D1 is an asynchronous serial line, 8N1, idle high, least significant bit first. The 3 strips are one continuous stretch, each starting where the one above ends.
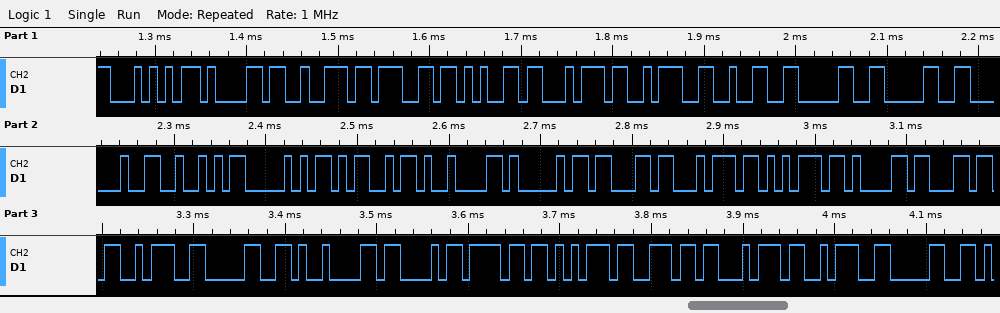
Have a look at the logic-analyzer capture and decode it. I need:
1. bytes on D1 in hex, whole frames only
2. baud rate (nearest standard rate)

54 61 72 67 65 74 3A 32 30 30 20 52 50 4D 09 41 63 74 75 61 6C 3A 30 09 43 6F 75 6E 74 3A 30
115200 baud
